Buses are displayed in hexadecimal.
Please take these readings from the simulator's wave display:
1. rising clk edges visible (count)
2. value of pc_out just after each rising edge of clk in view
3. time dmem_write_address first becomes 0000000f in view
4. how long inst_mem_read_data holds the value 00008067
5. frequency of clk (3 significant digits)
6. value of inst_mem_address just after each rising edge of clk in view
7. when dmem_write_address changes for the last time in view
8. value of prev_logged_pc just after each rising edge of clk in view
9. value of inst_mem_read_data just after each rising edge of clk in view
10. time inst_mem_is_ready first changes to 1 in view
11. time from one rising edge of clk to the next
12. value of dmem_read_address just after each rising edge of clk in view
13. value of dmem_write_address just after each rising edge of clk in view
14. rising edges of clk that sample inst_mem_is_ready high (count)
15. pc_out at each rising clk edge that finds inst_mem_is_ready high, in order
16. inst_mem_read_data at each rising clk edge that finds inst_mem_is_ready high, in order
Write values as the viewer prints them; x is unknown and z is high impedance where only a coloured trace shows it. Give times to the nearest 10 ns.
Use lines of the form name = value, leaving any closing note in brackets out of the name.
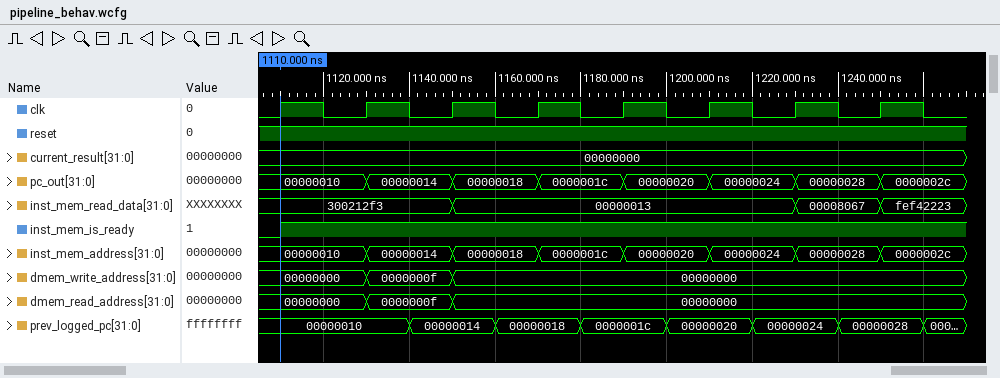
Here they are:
rising clk edges visible = 8
value of pc_out just after each rising edge of clk in view = 00000010, 00000014, 00000018, 0000001c, 00000020, 00000024, 00000028, 0000002c
time dmem_write_address first becomes 0000000f in view = 1130 ns
how long inst_mem_read_data holds the value 00008067 = 20 ns
frequency of clk = 50.0 MHz
value of inst_mem_address just after each rising edge of clk in view = 00000010, 00000014, 00000018, 0000001c, 00000020, 00000024, 00000028, 0000002c
when dmem_write_address changes for the last time in view = 1150 ns
value of prev_logged_pc just after each rising edge of clk in view = 00000010, 00000010, 00000014, 00000018, 0000001c, 00000020, 00000024, 00000028
value of inst_mem_read_data just after each rising edge of clk in view = 300212f3, 300212f3, 00000013, 00000013, 00000013, 00000013, 00008067, fef42223
time inst_mem_is_ready first changes to 1 in view = 1110 ns
time from one rising edge of clk to the next = 20 ns
value of dmem_read_address just after each rising edge of clk in view = 00000000, 0000000f, 00000000, 00000000, 00000000, 00000000, 00000000, 00000000
value of dmem_write_address just after each rising edge of clk in view = 00000000, 0000000f, 00000000, 00000000, 00000000, 00000000, 00000000, 00000000
rising edges of clk that sample inst_mem_is_ready high = 7
pc_out at each rising clk edge that finds inst_mem_is_ready high, in order = 00000010, 00000014, 00000018, 0000001c, 00000020, 00000024, 00000028
inst_mem_read_data at each rising clk edge that finds inst_mem_is_ready high, in order = 300212f3, 300212f3, 00000013, 00000013, 00000013, 00000013, 00008067
